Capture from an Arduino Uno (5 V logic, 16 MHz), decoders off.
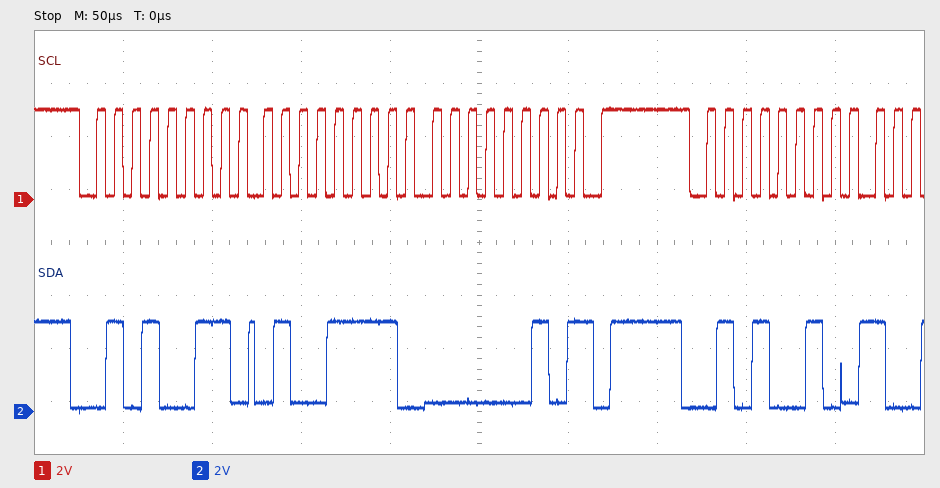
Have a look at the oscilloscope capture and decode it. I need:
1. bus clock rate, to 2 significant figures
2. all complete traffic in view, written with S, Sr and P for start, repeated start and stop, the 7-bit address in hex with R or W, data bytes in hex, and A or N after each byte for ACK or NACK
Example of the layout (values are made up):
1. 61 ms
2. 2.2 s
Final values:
1. 100 kHz
2. S 29R A 4F A 02 N P S 29W A
